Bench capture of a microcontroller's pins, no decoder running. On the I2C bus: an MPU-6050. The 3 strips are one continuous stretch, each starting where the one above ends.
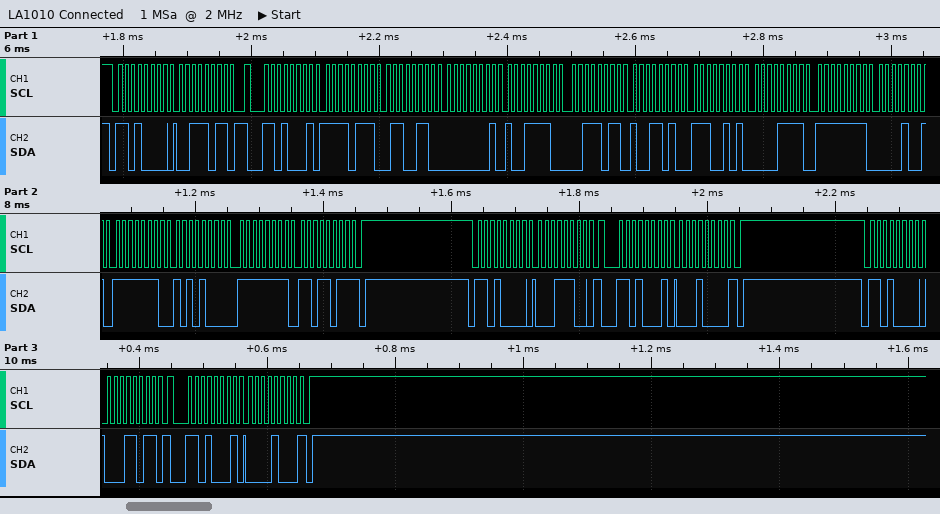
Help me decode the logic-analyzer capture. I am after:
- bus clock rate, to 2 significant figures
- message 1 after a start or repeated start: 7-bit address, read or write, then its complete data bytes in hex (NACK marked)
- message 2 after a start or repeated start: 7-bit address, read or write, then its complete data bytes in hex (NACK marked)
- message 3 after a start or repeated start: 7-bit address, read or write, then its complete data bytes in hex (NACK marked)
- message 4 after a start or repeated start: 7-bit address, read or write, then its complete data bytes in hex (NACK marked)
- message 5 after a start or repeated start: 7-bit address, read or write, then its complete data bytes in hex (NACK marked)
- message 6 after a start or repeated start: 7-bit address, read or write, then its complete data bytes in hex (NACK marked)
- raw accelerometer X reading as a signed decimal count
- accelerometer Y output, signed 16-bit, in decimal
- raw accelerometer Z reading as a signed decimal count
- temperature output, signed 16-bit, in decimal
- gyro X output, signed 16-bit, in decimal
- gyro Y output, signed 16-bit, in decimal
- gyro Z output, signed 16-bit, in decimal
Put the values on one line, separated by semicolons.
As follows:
100 kHz; 0x68 write: 3B; 0x68 read: F7 66 01 9E 3B 9A E5 0F FF 09 FE A8 FF DB NACK; 0x68 write: 1C; 0x68 read: 10 NACK; 0x68 write: 1B; 0x68 read: 08 NACK; -2202; 414; 15258; -6897; -247; -344; -37
